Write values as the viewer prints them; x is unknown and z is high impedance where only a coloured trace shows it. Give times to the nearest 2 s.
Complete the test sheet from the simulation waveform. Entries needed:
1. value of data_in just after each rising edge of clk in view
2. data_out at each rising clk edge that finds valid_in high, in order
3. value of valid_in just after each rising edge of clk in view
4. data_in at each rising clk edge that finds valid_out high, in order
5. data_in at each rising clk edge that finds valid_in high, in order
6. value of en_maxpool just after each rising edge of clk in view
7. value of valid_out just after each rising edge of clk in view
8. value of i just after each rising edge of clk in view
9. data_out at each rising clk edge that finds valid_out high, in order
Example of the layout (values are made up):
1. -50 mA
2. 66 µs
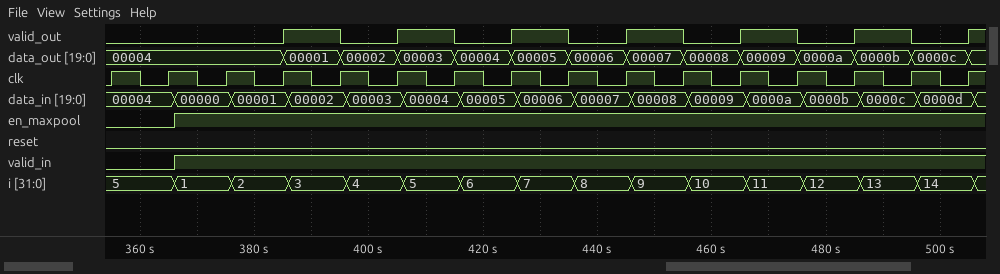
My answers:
1. 00004, 00004, 00000, 00001, 00002, 00003, 00004, 00005, 00006, 00007, 00008, 00009, 0000a, 0000b, 0000c, 0000d
2. 00004, 00004, 00001, 00002, 00003, 00004, 00005, 00006, 00007, 00008, 00009, 0000a, 0000b, 0000c
3. 0 0 1 1 1 1 1 1 1 1 1 1 1 1 1 1
4. 00002, 00004, 00006, 00008, 0000a, 0000c
5. 00000, 00001, 00002, 00003, 00004, 00005, 00006, 00007, 00008, 00009, 0000a, 0000b, 0000c, 0000d
6. 0 0 1 1 1 1 1 1 1 1 1 1 1 1 1 1
7. 0 0 0 1 0 1 0 1 0 1 0 1 0 1 0 1
8. 5, 5, 1, 2, 3, 4, 5, 6, 7, 8, 9, 10, 11, 12, 13, 14
9. 00001, 00003, 00005, 00007, 00009, 0000b
